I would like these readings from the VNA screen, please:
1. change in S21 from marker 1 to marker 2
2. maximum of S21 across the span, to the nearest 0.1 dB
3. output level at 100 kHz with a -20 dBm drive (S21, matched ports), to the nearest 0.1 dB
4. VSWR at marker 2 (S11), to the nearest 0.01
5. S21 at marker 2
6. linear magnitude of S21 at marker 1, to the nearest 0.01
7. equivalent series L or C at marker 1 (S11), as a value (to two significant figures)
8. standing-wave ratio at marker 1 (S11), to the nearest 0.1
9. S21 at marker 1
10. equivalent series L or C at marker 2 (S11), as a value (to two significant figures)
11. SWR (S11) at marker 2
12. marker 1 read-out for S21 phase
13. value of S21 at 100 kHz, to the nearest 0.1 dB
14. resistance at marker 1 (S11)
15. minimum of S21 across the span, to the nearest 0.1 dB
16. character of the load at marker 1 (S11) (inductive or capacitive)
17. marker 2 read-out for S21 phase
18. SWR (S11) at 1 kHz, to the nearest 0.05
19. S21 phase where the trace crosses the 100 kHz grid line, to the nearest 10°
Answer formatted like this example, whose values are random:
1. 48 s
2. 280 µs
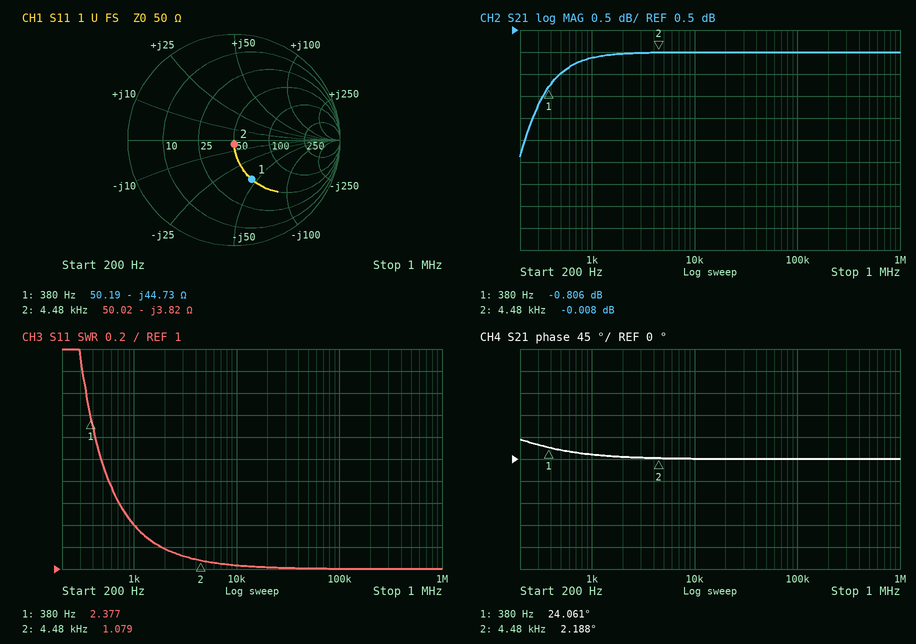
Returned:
1. 0.798 dB
2. 0.0 dB
3. -20.0 dBm
4. 1.08
5. -0.008 dB
6. 0.91
7. 9.4 µF
8. 2.4
9. -0.806 dB
10. 9.3 µF
11. 1.079
12. 24.061°
13. 0.0 dB
14. 50.19 Ω
15. -2.4 dB
16. capacitive
17. 2.188°
18. 1.40
19. 0°
